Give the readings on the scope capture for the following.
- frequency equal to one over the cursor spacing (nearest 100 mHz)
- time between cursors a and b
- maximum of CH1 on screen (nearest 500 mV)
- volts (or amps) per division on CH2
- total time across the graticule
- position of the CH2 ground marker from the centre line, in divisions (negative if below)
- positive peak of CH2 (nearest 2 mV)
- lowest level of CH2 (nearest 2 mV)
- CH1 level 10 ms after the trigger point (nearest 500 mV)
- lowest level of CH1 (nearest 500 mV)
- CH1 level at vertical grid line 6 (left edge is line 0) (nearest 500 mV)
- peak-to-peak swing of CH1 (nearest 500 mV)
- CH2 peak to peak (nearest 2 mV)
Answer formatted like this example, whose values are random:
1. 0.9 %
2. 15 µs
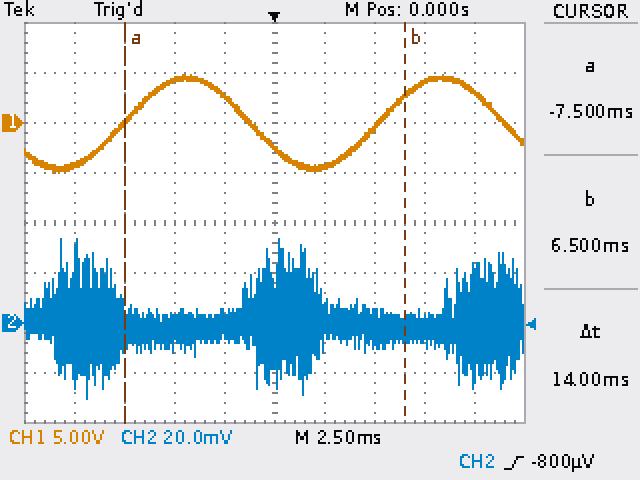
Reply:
1. 71.4 Hz
2. 14 ms
3. 5.0 V
4. 20 mV
5. 25 ms
6. -2.0 div
7. 34 mV
8. -30 mV
9. 3.0 V
10. -5.0 V
11. -4.5 V
12. 10.0 V
13. 64 mV
